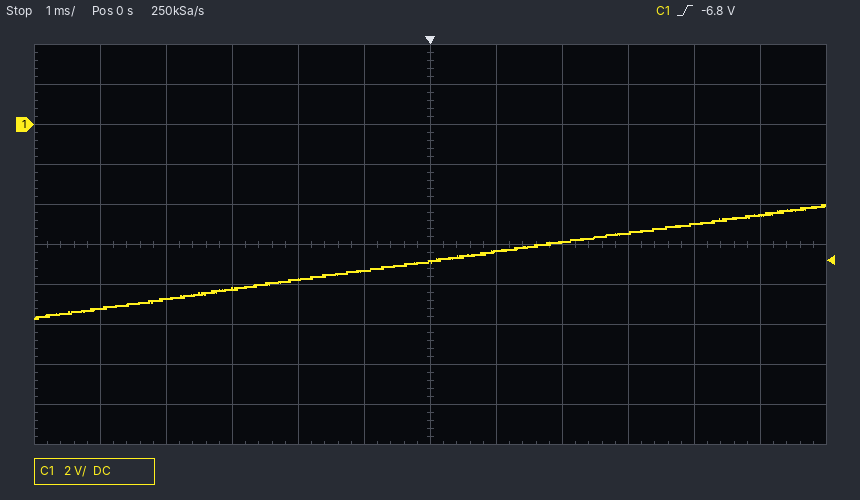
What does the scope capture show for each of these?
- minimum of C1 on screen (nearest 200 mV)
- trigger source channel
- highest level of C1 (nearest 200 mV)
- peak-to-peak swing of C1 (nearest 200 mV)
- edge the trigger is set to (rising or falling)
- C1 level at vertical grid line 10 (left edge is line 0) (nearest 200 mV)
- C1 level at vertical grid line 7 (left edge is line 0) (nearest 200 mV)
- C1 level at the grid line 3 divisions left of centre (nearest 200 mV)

-9.6 V
C1
-4.0 V
5.6 V
rising
-5.0 V
-6.4 V
-8.2 V
